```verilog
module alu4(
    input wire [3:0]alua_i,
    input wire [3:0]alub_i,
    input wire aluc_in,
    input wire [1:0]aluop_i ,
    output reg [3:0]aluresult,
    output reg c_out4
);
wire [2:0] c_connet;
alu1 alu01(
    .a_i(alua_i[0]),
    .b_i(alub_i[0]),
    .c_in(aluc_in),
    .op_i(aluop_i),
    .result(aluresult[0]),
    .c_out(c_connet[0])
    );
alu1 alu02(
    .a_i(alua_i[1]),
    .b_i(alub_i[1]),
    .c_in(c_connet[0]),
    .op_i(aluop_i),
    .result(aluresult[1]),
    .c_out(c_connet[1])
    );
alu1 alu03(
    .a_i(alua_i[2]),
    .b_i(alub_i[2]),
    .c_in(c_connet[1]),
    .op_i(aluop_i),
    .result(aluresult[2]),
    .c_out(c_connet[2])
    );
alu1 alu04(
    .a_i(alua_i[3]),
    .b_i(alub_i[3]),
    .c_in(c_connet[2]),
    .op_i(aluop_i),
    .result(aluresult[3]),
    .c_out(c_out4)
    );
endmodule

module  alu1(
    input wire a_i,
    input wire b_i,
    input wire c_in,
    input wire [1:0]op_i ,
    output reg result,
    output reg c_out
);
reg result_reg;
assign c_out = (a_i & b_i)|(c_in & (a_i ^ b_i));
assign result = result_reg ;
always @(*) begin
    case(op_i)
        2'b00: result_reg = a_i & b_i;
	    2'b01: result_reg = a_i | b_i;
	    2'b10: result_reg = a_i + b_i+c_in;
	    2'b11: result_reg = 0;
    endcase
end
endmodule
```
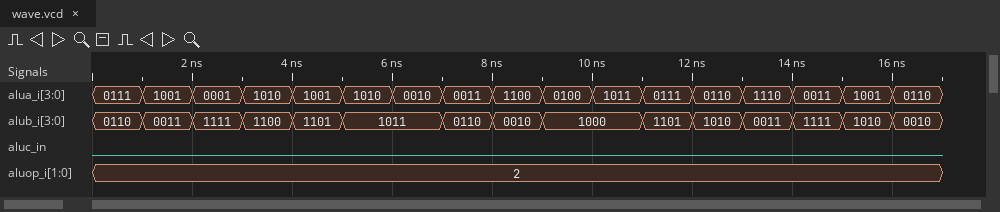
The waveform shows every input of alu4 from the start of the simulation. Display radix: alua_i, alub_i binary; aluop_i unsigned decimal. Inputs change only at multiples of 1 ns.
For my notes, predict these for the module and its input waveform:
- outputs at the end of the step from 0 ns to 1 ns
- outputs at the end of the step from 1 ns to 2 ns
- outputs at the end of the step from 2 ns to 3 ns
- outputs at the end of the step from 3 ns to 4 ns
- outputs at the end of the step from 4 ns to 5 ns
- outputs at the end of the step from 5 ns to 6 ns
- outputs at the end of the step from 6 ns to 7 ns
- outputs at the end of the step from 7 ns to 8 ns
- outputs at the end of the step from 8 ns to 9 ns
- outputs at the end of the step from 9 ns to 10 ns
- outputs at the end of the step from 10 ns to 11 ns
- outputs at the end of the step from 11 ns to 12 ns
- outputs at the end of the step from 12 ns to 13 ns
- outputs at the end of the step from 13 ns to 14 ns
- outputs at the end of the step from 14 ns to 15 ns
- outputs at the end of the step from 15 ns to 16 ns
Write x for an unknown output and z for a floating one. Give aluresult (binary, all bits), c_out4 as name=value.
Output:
aluresult=1101, c_out4=0
aluresult=1100, c_out4=0
aluresult=0000, c_out4=1
aluresult=0110, c_out4=1
aluresult=0110, c_out4=1
aluresult=0101, c_out4=1
aluresult=1101, c_out4=0
aluresult=1001, c_out4=0
aluresult=1110, c_out4=0
aluresult=1100, c_out4=0
aluresult=0011, c_out4=1
aluresult=0100, c_out4=1
aluresult=0000, c_out4=1
aluresult=0001, c_out4=1
aluresult=0010, c_out4=1
aluresult=0011, c_out4=1
